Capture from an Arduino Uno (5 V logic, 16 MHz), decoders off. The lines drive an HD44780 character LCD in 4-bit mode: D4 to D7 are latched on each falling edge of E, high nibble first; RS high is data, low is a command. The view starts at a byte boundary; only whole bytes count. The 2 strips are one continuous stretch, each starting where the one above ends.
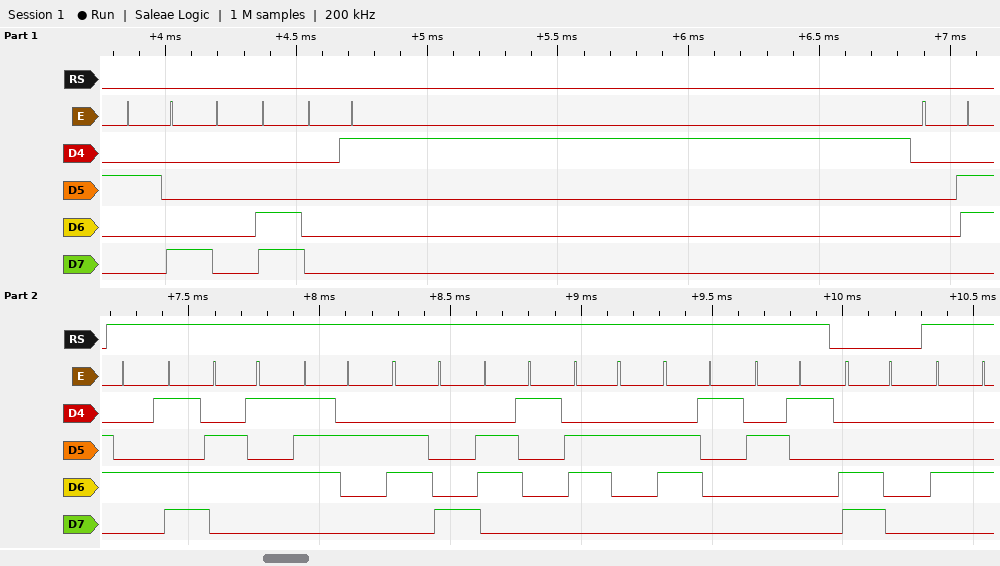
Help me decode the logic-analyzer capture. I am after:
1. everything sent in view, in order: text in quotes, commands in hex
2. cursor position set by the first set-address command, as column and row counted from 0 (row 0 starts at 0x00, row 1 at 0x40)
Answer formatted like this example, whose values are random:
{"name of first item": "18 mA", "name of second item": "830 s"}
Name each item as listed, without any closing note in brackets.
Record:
{"everything sent in view, in order: text in quotes, commands in hex": "0x28 0x0C 0x01 0x06 \"Merhaba!\" 0xC0 \"D\"", "cursor position set by the first set-address command, as column and row counted from 0": "column 0, row 1"}
